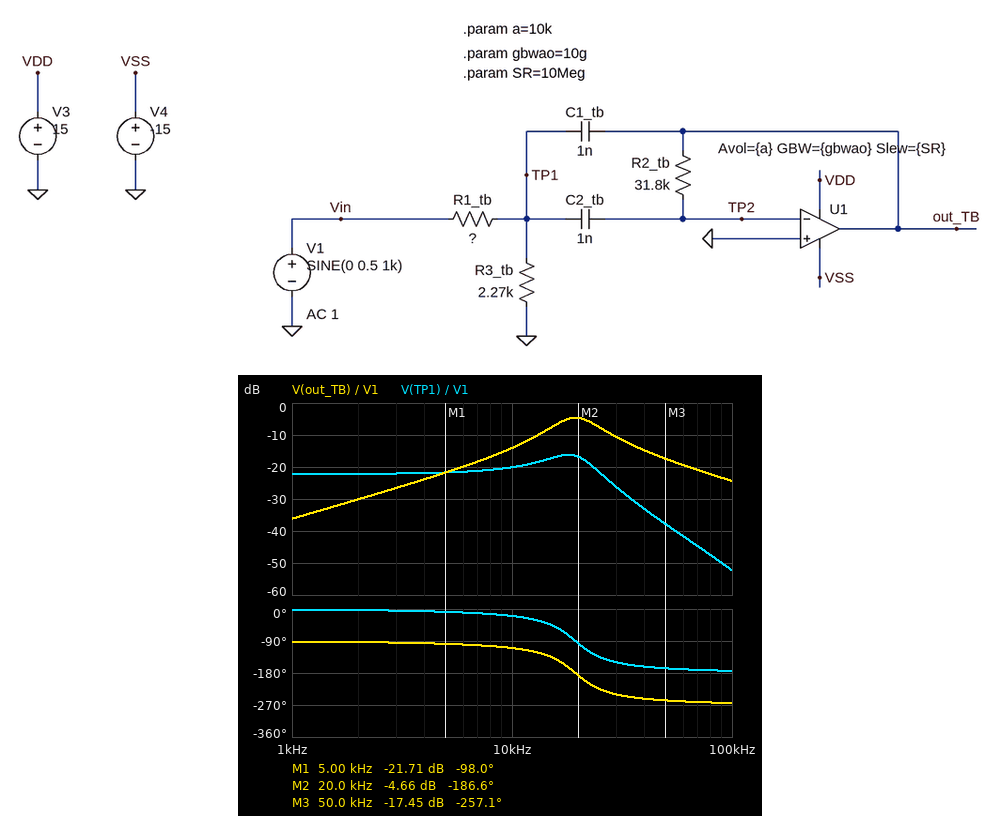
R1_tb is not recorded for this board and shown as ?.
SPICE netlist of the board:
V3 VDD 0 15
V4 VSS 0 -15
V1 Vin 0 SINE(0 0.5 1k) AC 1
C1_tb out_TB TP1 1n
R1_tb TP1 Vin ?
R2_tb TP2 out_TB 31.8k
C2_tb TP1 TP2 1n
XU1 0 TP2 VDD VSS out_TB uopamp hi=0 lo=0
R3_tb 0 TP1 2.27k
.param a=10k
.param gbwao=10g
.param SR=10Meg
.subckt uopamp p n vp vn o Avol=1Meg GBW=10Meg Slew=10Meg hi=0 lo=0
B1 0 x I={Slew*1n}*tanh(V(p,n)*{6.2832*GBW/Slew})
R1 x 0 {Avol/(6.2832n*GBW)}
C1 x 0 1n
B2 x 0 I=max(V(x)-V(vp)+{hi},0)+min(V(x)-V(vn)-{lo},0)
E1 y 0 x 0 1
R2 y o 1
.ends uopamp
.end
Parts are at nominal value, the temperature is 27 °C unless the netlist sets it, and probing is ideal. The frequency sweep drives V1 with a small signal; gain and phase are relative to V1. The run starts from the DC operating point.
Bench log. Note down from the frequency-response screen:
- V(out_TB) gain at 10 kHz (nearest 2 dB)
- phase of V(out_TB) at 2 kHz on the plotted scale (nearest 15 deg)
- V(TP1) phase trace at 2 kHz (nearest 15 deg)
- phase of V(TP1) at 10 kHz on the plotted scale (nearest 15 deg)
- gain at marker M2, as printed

-14 dB
-90 deg
0 deg
-15 deg
-4.66 dB
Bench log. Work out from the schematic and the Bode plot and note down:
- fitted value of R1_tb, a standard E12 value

27 kΩ
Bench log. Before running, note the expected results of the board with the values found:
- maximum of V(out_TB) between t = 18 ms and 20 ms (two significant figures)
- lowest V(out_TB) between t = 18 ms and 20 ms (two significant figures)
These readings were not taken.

7.8 mV
-7.8 mV
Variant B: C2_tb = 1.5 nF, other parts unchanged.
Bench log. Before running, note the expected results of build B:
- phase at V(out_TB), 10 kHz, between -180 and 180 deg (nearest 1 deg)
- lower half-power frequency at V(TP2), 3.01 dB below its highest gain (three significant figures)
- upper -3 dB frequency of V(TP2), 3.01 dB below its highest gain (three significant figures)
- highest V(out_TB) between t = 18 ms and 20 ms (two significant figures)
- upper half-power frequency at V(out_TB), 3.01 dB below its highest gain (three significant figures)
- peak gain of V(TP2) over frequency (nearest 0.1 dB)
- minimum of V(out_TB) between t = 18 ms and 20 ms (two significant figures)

-119 deg
13.6 kHz
26.4 kHz
12 mV
20.5 kHz
-58.7 dB
-12 mV
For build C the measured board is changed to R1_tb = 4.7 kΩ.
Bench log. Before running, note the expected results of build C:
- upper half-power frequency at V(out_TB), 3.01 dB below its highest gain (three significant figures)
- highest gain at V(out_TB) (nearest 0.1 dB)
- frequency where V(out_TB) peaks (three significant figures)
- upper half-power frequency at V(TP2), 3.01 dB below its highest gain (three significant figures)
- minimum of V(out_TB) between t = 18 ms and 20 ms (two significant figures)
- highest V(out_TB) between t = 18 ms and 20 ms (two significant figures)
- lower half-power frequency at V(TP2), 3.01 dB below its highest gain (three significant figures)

28.2 kHz
10.6 dB
22.7 kHz
32.8 kHz
-33 mV
33 mV
19.7 kHz
